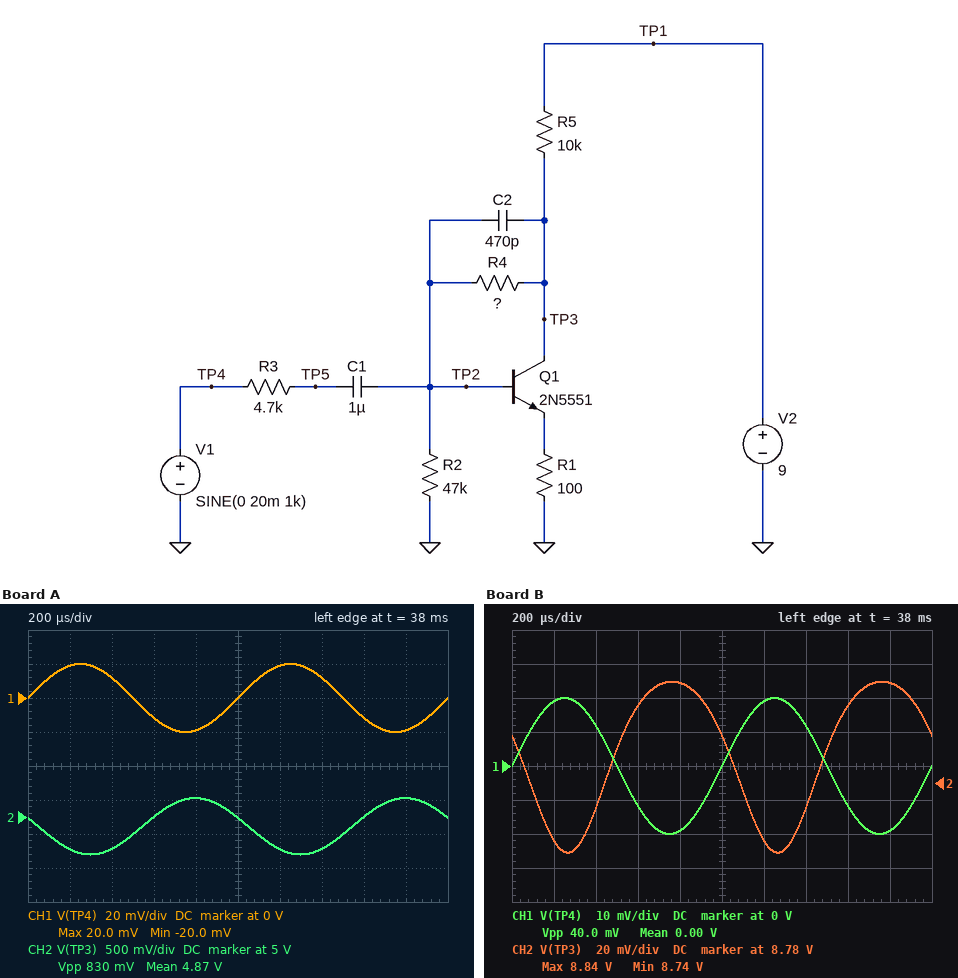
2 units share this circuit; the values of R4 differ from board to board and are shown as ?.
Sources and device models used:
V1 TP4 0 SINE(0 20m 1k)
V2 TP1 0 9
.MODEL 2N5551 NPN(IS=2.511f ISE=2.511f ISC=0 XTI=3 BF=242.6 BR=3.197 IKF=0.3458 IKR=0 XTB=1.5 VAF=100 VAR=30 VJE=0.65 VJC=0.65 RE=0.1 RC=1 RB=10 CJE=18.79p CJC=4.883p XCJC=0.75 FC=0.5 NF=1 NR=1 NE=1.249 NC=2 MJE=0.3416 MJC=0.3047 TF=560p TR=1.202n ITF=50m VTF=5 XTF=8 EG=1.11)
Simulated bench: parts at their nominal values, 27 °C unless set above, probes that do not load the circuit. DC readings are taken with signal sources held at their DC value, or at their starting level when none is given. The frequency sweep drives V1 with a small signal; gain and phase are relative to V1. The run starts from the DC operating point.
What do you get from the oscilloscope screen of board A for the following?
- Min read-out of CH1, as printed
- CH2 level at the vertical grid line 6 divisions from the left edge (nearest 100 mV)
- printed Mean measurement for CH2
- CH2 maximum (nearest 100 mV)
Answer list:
-20.0 mV
4.5 V
4.87 V
5.3 V
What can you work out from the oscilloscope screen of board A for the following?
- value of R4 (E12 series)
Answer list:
220 kΩ
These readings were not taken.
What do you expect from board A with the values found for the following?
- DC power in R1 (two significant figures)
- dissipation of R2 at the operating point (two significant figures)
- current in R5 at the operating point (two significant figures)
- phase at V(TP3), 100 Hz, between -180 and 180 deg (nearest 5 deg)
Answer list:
16 µW
11 µW
410 µA
-170 deg
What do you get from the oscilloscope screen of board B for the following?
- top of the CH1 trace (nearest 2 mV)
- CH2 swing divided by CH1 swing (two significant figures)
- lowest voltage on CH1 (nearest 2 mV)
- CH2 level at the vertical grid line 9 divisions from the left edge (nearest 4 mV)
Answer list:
20 mV
2.5
-20 mV
8.840 V
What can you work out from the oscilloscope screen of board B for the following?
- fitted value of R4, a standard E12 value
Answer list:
680 kΩ
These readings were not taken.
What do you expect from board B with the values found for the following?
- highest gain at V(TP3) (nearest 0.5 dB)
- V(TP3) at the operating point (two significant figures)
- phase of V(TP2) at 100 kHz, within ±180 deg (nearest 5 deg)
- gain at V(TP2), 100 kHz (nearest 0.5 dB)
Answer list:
7.5 dB
8.8 V
-15 deg
-9.0 dB
